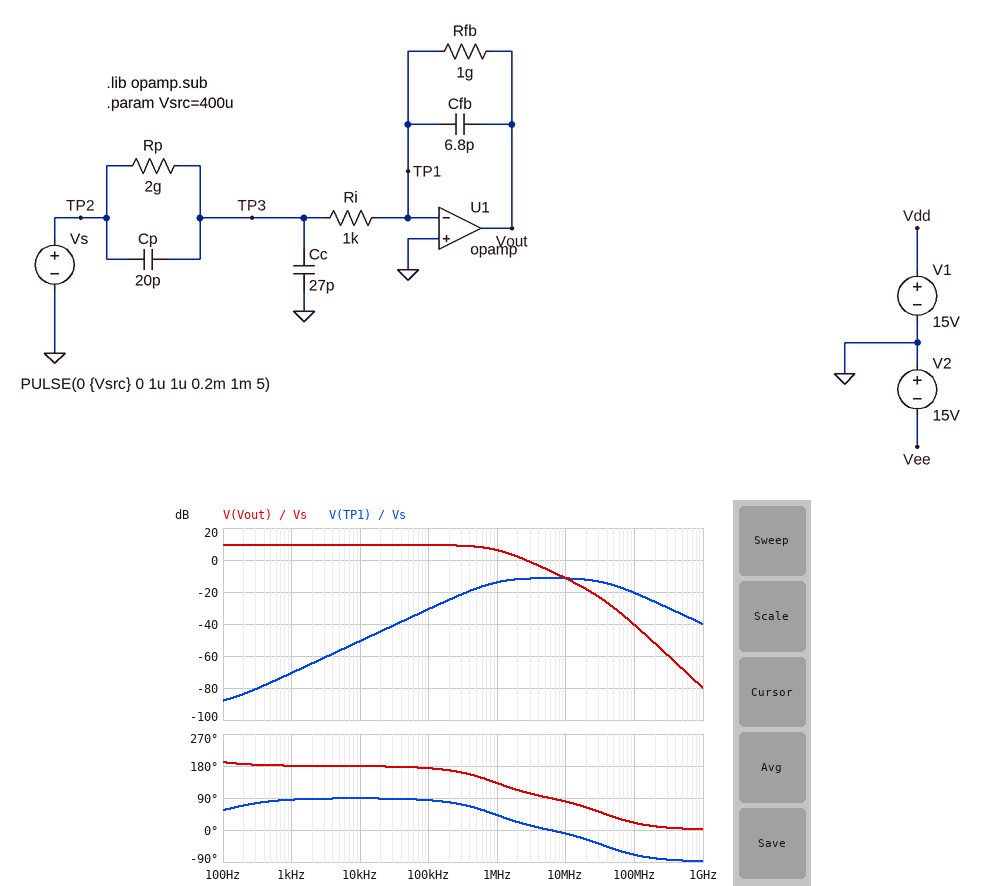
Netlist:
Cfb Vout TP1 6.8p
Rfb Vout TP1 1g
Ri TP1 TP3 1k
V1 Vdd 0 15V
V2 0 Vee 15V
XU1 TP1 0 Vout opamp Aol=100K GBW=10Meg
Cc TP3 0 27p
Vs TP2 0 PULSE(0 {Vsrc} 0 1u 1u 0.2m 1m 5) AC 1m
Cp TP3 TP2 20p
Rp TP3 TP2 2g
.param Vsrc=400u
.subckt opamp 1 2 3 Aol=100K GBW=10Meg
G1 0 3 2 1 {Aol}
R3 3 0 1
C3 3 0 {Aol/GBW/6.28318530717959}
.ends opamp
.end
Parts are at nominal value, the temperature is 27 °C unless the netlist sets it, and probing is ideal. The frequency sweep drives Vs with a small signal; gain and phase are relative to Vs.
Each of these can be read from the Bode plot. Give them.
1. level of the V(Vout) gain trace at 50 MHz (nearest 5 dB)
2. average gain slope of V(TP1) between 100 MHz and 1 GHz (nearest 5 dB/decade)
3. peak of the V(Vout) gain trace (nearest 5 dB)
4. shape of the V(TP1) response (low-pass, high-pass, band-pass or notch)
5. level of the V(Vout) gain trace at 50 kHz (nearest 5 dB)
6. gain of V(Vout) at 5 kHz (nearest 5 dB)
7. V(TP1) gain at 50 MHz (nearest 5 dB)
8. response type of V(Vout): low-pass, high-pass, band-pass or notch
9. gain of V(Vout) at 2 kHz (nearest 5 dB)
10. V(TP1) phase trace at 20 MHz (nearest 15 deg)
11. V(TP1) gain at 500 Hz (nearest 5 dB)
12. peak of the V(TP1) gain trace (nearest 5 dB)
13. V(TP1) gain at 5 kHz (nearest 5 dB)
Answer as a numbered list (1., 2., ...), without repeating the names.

1. -30 dB
2. -20 dB/decade
3. 10 dB
4. band-pass
5. 10 dB
6. 10 dB
7. -15 dB
8. low-pass
9. 10 dB
10. -30 deg
11. -75 dB
12. -10 dB
13. -55 dB
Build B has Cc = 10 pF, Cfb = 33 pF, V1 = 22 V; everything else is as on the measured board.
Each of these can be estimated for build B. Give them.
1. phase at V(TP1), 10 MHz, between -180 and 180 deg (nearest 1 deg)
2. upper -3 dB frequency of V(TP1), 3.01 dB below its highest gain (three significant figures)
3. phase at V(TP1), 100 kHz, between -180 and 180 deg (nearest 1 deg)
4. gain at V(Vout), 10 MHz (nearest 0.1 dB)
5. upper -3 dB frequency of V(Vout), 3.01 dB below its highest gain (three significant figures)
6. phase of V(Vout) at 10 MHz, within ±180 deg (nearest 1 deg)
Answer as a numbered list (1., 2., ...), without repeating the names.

1. -13 deg
2. 22.5 MHz
3. 88 deg
4. -16.2 dB
5. 3.02 MHz
6. 77 deg
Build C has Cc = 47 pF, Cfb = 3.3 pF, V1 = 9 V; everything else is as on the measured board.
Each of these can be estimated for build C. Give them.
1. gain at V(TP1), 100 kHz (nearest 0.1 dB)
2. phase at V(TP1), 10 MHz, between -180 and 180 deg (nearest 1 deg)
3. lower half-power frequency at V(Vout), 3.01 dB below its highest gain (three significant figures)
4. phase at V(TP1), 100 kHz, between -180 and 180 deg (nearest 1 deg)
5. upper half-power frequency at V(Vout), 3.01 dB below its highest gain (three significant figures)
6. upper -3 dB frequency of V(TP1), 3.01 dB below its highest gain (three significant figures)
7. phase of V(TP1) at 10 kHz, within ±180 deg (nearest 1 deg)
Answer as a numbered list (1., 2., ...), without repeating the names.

1. -24.6 dB
2. -7 deg
3. 47.9 Hz
4. 76 deg
5. 395 kHz
6. 61.0 MHz
7. 88 deg
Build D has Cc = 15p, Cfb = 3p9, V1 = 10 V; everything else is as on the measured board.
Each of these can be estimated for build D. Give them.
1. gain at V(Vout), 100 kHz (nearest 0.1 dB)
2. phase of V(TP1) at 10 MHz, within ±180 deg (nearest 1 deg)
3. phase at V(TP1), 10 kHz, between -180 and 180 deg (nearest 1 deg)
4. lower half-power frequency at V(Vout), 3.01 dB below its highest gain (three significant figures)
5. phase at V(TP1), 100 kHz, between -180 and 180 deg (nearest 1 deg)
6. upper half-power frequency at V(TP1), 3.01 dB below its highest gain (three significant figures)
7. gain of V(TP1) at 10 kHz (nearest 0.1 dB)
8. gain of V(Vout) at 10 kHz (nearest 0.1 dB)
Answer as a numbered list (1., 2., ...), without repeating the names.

1. 14.1 dB
2. -6 deg
3. 89 deg
4. 40.4 Hz
5. 83 deg
6. 56.2 MHz
7. -45.8 dB
8. 14.2 dB
